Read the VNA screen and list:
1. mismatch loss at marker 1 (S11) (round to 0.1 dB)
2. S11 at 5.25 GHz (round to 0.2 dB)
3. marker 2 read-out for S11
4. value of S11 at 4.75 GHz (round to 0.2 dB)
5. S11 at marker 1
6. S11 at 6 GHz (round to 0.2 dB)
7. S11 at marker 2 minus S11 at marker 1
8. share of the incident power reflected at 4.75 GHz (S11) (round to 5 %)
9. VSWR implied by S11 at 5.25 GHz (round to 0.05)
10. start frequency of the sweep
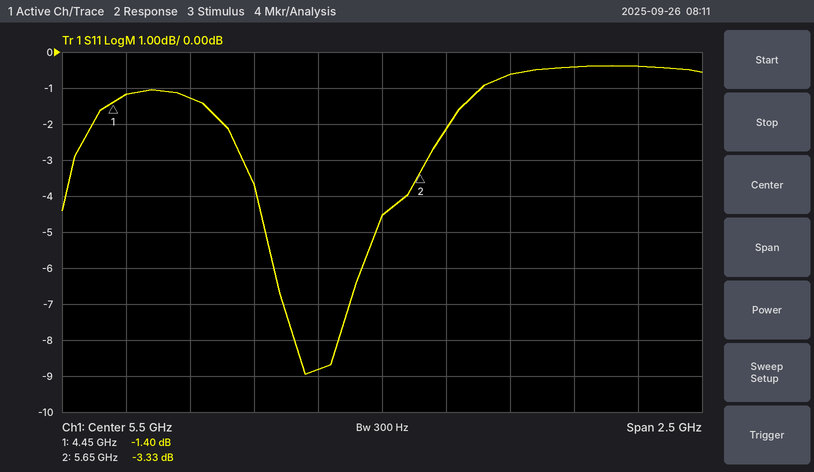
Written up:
5.6 dB
-8.8 dB
-3.33 dB
-1.2 dB
-1.40 dB
-0.6 dB
-1.93 dB
75 %
2.15
4.25 GHz
